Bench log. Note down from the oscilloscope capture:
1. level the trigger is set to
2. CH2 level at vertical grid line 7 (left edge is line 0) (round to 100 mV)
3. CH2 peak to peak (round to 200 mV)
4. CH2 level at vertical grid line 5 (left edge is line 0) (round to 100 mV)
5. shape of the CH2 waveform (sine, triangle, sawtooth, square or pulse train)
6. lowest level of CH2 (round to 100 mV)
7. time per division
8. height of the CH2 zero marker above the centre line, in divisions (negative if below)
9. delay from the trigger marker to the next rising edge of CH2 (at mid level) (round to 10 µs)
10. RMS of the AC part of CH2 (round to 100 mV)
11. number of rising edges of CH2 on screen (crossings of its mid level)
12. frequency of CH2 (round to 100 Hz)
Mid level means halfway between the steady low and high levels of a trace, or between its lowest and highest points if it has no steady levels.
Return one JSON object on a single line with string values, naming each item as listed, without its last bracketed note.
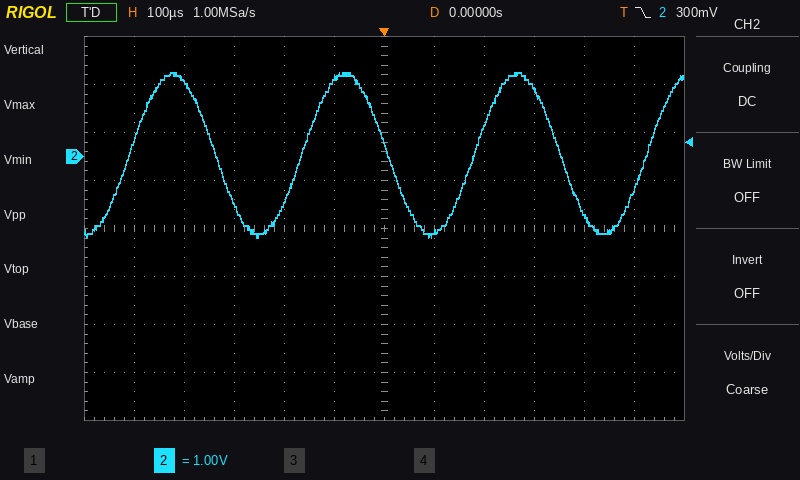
{"level the trigger is set to": "300 mV", "CH2 level at vertical grid line 7 (left edge is line 0)": "-1.6 V", "CH2 peak to peak": "3.4 V", "CH2 level at vertical grid line 5 (left edge is line 0)": "1.6 V", "shape of the CH2 waveform": "sine", "lowest level of CH2": "-1.7 V", "time per division": "100 µs", "height of the CH2 zero marker above the centre line, in divisions": "+1.5 div", "delay from the trigger marker to the next rising edge of CH2 (at mid level)": "180 µs", "RMS of the AC part of CH2": "1.2 V", "number of rising edges of CH2 on screen": "4", "frequency of CH2": "2.9 kHz"}
